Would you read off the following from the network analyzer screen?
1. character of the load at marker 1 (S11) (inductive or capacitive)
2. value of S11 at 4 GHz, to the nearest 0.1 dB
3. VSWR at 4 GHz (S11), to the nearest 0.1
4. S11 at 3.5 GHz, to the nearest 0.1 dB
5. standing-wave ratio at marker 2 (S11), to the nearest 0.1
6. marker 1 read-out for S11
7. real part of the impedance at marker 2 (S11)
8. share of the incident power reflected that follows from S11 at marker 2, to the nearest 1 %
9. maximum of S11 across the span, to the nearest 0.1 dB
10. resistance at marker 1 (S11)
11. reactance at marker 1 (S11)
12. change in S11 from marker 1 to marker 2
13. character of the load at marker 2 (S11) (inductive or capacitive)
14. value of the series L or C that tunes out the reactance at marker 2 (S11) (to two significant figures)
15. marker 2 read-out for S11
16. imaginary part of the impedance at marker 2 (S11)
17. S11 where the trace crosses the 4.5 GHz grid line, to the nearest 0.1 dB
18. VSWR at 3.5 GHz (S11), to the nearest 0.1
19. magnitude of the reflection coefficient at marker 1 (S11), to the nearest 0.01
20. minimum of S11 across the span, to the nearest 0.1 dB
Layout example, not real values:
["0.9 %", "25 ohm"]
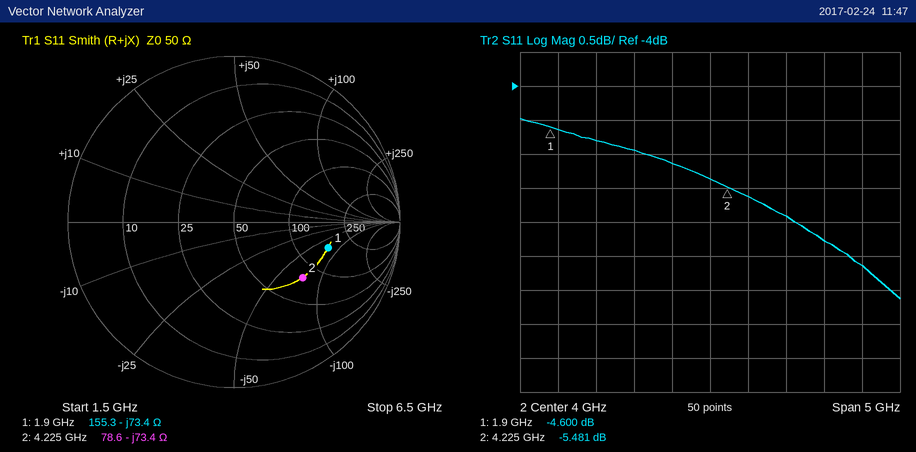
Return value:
["capacitive", "-5.4 dB", "3.3", "-5.1 dB", "3.3", "-4.600 dB", "78.6 Ω", "28 %", "-4.5 dB", "155.3 Ω", "-73.4 Ω", "-0.881 dB", "capacitive", "2.8 nH", "-5.481 dB", "-73.4 Ω", "-5.6 dB", "3.5", "0.59", "-7.1 dB"]
